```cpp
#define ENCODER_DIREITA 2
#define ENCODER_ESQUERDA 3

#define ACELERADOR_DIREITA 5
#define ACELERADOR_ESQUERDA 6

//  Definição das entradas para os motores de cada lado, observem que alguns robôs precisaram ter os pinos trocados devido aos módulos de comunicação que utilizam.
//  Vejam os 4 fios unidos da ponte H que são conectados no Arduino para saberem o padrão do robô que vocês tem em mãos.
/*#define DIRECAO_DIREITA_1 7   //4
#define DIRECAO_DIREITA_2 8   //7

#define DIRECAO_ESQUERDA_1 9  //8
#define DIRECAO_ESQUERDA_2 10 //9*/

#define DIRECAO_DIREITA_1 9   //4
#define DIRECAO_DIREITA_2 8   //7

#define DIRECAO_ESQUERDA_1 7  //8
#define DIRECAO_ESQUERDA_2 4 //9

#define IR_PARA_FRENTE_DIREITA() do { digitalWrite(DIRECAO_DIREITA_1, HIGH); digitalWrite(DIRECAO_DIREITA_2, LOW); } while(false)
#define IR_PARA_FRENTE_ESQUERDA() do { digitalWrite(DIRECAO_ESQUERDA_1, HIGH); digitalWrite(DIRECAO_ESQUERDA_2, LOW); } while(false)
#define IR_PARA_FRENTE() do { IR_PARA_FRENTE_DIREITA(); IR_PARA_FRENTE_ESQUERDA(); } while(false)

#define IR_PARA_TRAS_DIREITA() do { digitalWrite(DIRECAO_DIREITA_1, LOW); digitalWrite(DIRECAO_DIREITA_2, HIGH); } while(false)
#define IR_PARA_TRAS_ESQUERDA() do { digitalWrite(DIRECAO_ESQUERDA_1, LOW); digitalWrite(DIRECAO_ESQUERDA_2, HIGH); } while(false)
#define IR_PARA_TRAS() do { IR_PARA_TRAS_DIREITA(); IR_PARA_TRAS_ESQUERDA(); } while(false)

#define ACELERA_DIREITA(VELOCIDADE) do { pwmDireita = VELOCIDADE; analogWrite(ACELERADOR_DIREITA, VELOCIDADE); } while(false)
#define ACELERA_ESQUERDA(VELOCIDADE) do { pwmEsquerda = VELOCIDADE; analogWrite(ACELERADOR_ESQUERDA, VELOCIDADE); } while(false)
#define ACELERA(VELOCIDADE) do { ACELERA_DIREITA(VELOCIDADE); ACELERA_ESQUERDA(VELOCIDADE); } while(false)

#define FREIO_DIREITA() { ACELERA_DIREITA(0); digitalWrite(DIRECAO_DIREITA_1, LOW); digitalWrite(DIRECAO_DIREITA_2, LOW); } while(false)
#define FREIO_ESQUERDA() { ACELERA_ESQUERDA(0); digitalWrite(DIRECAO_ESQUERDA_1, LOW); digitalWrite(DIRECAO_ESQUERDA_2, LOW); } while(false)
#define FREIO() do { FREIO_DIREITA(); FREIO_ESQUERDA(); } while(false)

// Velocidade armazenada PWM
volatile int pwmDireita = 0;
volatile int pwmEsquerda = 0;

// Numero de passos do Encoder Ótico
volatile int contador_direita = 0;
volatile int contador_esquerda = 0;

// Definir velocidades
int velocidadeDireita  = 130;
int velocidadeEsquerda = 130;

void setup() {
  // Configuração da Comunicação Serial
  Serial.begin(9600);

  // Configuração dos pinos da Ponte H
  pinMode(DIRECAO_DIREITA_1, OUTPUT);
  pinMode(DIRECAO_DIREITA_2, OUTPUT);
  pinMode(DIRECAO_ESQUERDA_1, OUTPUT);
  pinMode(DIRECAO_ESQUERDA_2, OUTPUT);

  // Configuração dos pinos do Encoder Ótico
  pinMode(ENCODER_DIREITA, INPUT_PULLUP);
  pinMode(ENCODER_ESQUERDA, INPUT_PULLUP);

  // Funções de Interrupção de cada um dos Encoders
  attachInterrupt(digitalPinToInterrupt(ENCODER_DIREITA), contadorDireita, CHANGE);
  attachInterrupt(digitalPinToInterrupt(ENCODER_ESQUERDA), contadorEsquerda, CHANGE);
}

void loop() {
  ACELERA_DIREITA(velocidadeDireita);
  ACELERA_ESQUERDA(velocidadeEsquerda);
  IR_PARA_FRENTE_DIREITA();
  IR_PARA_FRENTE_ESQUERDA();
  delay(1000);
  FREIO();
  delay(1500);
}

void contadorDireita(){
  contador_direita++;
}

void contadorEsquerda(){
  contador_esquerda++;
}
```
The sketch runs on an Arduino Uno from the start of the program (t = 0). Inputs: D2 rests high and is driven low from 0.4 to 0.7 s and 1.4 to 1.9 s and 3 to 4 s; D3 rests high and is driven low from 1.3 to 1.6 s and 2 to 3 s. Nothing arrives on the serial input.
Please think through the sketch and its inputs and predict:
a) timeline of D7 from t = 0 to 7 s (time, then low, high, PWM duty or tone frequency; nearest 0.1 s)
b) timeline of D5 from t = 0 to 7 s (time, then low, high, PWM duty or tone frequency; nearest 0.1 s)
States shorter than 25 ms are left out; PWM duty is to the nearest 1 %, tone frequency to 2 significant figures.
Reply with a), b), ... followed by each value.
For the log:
a) 0 s high; 1 s low; 2.5 s high; 3.5 s low; 5 s high; 6 s low
b) 0 s PWM 51 %; 1 s low; 2.5 s PWM 51 %; 3.5 s low; 5 s PWM 51 %; 6 s low
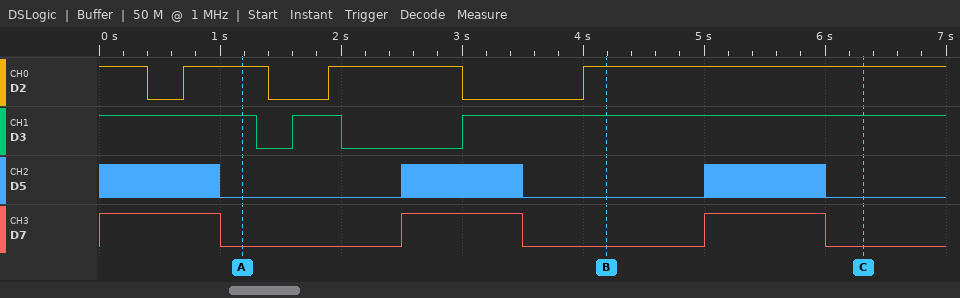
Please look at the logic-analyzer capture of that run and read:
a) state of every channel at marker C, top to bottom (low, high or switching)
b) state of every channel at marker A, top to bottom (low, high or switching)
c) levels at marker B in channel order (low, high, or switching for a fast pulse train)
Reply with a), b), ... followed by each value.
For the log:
a) D2 high, D3 high, D5 low, D7 low
b) D2 high, D3 high, D5 low, D7 low
c) D2 high, D3 high, D5 low, D7 low
